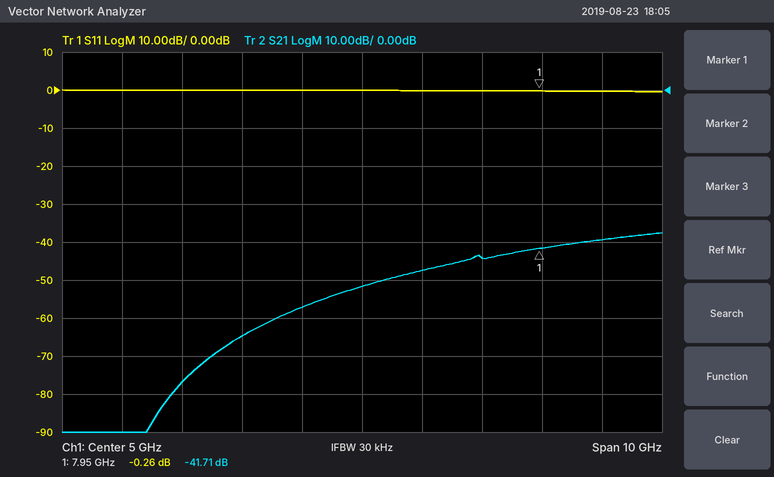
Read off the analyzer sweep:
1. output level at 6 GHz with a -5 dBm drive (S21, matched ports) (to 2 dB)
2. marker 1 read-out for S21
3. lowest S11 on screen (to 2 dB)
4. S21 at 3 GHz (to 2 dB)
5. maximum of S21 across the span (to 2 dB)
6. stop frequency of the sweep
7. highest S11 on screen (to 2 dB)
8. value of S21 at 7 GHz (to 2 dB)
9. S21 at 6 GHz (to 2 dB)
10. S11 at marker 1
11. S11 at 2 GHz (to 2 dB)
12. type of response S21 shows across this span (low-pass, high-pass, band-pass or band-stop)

-52 dBm
-41.71 dB
0 dB
-64 dB
-38 dB
10 GHz
0 dB
-44 dB
-48 dB
-0.26 dB
0 dB
high-pass
